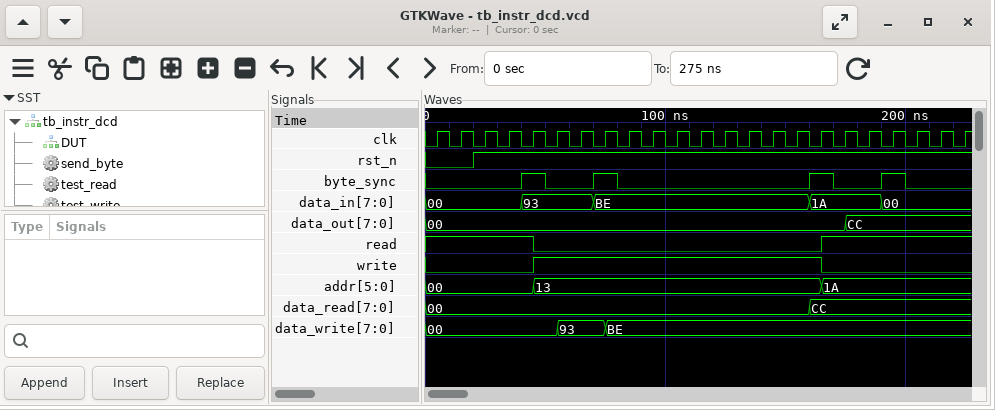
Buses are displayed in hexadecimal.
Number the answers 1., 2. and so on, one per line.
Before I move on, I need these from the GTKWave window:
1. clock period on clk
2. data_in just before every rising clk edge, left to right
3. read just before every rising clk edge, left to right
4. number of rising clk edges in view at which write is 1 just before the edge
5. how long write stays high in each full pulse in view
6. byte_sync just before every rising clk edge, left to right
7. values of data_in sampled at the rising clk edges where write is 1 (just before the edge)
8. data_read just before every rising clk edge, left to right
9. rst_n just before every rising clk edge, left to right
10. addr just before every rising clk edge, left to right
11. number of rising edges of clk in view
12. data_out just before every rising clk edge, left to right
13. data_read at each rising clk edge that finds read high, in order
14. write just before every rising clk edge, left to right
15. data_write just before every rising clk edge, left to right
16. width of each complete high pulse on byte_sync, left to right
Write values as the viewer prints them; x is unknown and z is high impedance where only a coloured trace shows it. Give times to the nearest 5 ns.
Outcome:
1. 10 ns
2. 00, 00, 00, 00, 93, 93, 93, BE, BE, BE, BE, BE, BE, BE, BE, BE, 1A, 1A, 1A, 00, 00, 00, 00
3. 1 1 1 1 1 0 0 0 0 0 0 0 0 0 0 0 0 1 1 1 1 1 1
4. 12
5. 120 ns
6. 0 0 0 0 1 0 0 1 0 0 0 0 0 0 0 0 1 0 0 1 0 0 0
7. 93, 93, BE, BE, BE, BE, BE, BE, BE, BE, BE, 1A
8. 00, 00, 00, 00, 00, 00, 00, 00, 00, 00, 00, 00, 00, 00, 00, 00, CC, CC, CC, CC, CC, CC, CC
9. 0 0 1 1 1 1 1 1 1 1 1 1 1 1 1 1 1 1 1 1 1 1 1
10. 00, 00, 00, 00, 00, 13, 13, 13, 13, 13, 13, 13, 13, 13, 13, 13, 13, 1A, 1A, 1A, 1A, 1A, 1A
11. 23
12. 00, 00, 00, 00, 00, 00, 00, 00, 00, 00, 00, 00, 00, 00, 00, 00, 00, 00, CC, CC, CC, CC, CC
13. 00, 00, 00, 00, 00, CC, CC, CC, CC, CC, CC
14. 0 0 0 0 0 1 1 1 1 1 1 1 1 1 1 1 1 0 0 0 0 0 0
15. 00, 00, 00, 00, 00, 00, 93, 93, BE, BE, BE, BE, BE, BE, BE, BE, BE, BE, BE, BE, BE, BE, BE
16. 10 ns, 10 ns, 10 ns, 10 ns
